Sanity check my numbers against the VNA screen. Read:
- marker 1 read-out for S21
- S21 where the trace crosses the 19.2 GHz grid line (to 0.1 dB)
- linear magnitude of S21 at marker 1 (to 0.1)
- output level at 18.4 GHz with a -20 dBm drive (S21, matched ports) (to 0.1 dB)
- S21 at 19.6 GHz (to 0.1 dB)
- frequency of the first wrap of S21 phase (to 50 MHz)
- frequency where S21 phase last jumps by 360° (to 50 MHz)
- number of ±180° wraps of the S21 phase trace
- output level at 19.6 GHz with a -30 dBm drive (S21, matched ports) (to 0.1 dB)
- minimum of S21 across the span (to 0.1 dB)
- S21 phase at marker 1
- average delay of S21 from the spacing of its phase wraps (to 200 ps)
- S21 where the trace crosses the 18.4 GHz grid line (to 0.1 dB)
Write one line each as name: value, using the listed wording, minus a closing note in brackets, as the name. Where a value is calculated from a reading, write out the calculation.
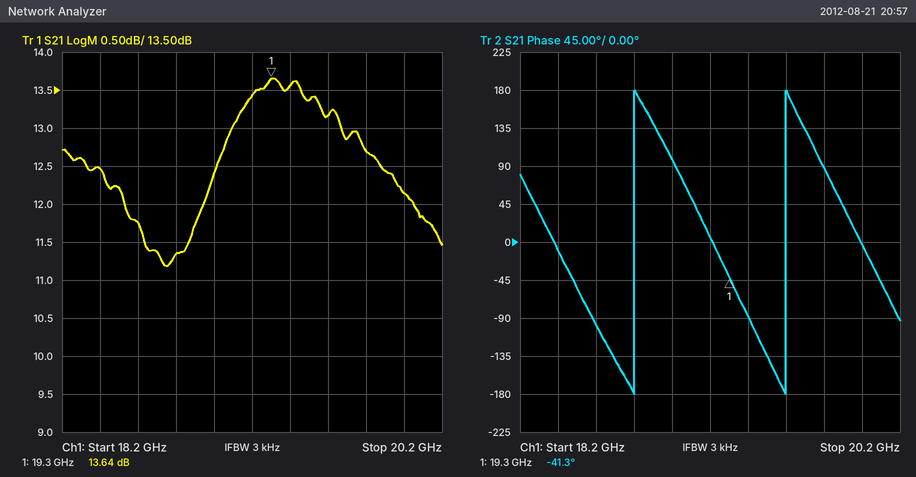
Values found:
marker 1 read-out for S21: 13.64 dB
S21 where the trace crosses the 19.2 GHz grid line: 13.4 dB
linear magnitude of S21 at marker 1: 10^(13.64/20) ≈ 4.8
output level at 18.4 GHz with a -20 dBm drive (S21, matched ports): -20 dBm + (12.5 dB) = -7.5 dBm
S21 at 19.6 GHz: 13.2 dB
frequency of the first wrap of S21 phase: 18.80 GHz
frequency where S21 phase last jumps by 360°: 19.60 GHz
number of ±180° wraps of the S21 phase trace: 2
output level at 19.6 GHz with a -30 dBm drive (S21, matched ports): -30 dBm + (13.2 dB) = -16.8 dBm
minimum of S21 across the span: 11.2 dB
S21 phase at marker 1: -41.3°
average delay of S21 from the spacing of its phase wraps: 1 cycle / (19.60 GHz − 18.80 GHz) ≈ 1.2 ns
S21 where the trace crosses the 18.4 GHz grid line: 12.5 dB
